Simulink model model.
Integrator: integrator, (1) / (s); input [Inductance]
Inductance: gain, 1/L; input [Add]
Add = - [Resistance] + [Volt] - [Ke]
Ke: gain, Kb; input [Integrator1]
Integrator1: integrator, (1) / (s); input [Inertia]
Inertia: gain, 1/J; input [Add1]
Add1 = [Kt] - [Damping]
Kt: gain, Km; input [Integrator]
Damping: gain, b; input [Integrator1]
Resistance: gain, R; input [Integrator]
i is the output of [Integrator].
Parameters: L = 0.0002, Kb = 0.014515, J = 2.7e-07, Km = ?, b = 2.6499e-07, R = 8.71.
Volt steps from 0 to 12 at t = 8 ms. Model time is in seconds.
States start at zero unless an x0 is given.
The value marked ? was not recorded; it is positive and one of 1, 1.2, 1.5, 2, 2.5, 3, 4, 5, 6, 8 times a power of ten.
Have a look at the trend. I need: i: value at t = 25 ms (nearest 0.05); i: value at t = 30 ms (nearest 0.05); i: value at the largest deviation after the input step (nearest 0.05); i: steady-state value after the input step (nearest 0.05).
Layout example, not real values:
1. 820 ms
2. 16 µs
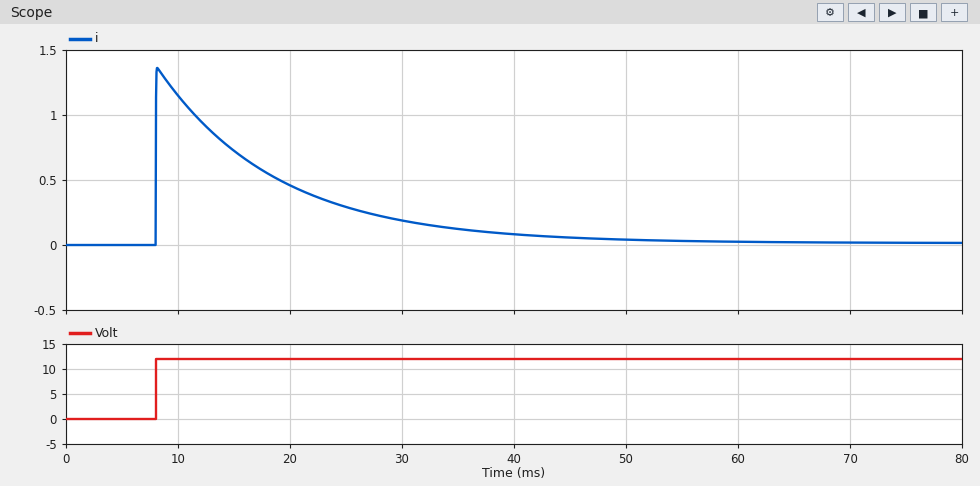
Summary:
1. 0.30
2. 0.20
3. 1.35
4. 0.00
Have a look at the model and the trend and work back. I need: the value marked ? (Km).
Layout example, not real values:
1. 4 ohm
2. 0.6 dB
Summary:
1. 0.015
